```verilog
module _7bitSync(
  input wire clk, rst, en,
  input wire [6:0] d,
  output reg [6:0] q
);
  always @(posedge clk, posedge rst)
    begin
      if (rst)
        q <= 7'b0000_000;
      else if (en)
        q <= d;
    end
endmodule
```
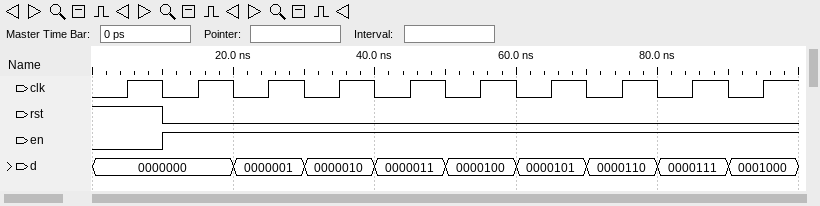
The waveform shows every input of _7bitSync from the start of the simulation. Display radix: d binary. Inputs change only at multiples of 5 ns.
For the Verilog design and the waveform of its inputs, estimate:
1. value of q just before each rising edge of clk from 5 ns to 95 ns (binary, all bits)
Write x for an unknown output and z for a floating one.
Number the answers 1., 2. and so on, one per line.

1. 0000000, 0000000, 0000000, 0000001, 0000010, 0000011, 0000100, 0000101, 0000110, 0000111
